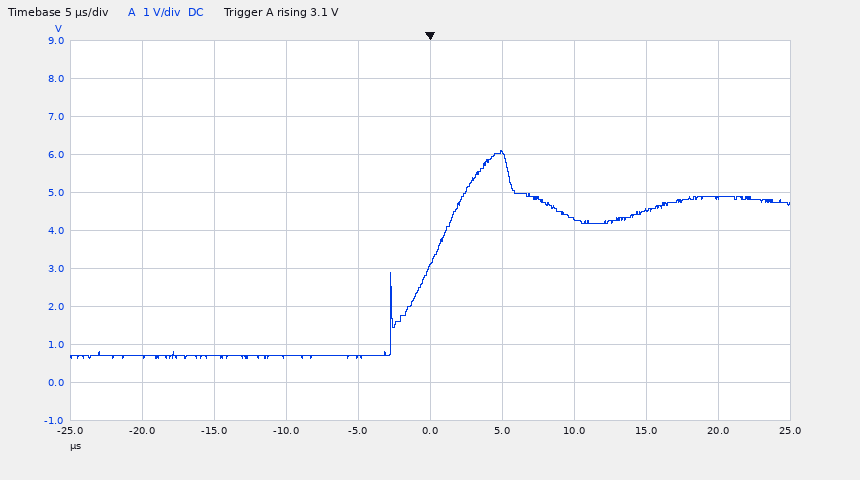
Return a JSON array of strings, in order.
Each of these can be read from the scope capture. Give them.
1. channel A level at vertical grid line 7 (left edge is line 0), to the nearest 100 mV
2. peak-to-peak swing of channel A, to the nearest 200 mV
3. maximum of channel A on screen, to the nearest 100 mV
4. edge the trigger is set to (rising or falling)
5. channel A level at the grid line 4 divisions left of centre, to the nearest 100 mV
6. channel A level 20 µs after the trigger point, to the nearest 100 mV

["4.3 V", "5.4 V", "6.1 V", "rising", "700 mV", "4.9 V"]
